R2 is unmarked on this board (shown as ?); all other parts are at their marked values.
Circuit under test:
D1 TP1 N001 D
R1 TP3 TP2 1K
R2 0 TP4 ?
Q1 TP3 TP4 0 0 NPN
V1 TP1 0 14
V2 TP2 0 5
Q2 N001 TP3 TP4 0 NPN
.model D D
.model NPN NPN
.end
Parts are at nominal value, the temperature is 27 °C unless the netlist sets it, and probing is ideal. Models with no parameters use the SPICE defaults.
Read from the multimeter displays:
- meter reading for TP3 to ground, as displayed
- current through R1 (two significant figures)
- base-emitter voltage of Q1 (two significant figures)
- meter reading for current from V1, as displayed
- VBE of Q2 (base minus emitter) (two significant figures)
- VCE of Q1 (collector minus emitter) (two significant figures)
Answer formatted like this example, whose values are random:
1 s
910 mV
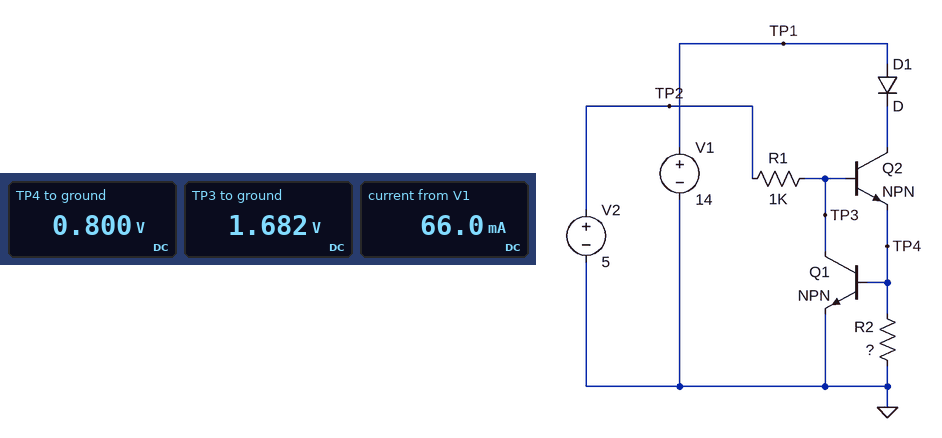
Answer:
1.682 V
3.3 mA
800 mV
66.0 mA
880 mV
1.7 V
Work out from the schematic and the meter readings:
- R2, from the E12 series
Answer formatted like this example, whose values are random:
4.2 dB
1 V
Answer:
12 Ω
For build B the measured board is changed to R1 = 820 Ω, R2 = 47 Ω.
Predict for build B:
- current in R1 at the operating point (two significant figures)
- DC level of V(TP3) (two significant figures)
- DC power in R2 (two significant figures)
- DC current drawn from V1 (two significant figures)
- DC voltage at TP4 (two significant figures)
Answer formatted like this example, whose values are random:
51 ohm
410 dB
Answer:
4.1 mA
1.7 V
14 mW
17 mA
810 mV
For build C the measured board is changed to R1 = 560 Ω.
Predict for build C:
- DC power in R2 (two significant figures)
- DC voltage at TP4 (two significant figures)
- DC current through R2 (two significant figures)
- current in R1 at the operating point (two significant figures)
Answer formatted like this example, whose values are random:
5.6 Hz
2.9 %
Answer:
56 mW
820 mV
68 mA
5.9 mA
